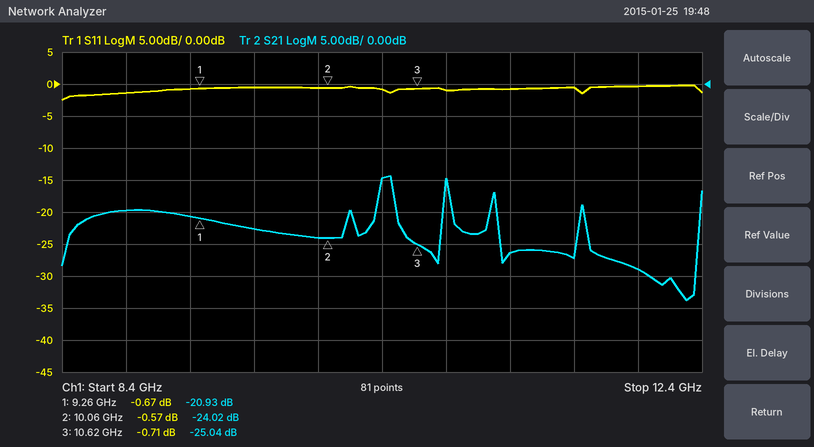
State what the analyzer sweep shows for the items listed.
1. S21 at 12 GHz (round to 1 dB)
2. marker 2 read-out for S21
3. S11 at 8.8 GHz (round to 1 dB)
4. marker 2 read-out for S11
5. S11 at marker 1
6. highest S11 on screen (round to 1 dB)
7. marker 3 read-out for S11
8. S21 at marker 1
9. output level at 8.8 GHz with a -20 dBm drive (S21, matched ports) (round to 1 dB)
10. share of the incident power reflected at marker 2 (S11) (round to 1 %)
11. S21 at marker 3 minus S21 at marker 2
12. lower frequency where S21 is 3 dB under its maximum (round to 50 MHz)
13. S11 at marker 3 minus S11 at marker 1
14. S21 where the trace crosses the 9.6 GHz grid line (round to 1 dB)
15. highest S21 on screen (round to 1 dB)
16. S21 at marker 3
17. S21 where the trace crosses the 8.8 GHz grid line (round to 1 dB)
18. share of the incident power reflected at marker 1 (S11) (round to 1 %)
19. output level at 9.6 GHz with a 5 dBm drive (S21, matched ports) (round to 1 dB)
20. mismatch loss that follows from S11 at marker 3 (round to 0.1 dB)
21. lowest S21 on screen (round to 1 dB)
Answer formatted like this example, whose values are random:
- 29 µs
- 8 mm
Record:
- -29 dB
- -24.02 dB
- -1 dB
- -0.57 dB
- -0.67 dB
- 0 dB
- -0.71 dB
- -20.93 dB
- -40 dBm
- 88 %
- -1.02 dB
- 10.40 GHz
- -0.04 dB
- -23 dB
- -14 dB
- -25.04 dB
- -20 dB
- 86 %
- -18 dBm
- 8.2 dB
- -34 dB
